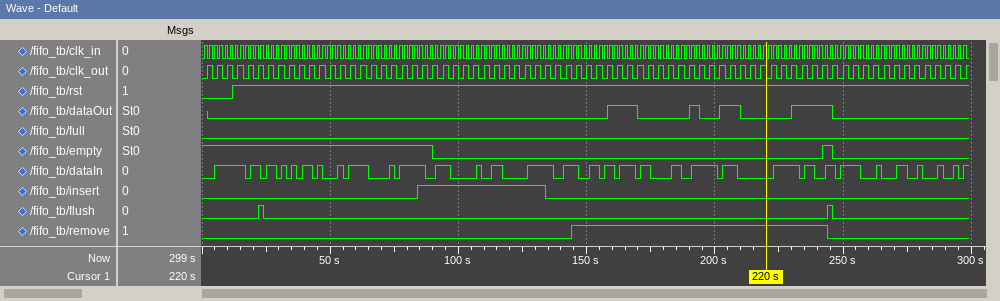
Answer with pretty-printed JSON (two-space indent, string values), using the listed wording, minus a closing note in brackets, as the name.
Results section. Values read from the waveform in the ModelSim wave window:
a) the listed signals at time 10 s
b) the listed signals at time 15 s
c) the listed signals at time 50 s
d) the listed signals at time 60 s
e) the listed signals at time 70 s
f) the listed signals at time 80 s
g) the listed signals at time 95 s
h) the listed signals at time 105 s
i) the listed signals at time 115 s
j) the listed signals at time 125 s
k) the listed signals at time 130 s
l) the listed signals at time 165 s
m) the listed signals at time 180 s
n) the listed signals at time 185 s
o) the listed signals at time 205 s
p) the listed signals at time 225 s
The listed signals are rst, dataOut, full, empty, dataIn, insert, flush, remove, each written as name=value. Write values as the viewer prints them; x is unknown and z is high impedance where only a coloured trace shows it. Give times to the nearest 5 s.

{
  "the listed signals at time 10 s": "rst=0, dataOut=0, full=0, empty=1, dataIn=1, insert=0, flush=0, remove=0",
  "the listed signals at time 15 s": "rst=1, dataOut=0, full=0, empty=1, dataIn=1, insert=0, flush=0, remove=0",
  "the listed signals at time 50 s": "rst=1, dataOut=0, full=0, empty=1, dataIn=0, insert=0, flush=0, remove=0",
  "the listed signals at time 60 s": "rst=1, dataOut=0, full=0, empty=1, dataIn=1, insert=0, flush=0, remove=0",
  "the listed signals at time 70 s": "rst=1, dataOut=0, full=0, empty=1, dataIn=0, insert=0, flush=0, remove=0",
  "the listed signals at time 80 s": "rst=1, dataOut=0, full=0, empty=1, dataIn=1, insert=0, flush=0, remove=0",
  "the listed signals at time 95 s": "rst=1, dataOut=0, full=0, empty=0, dataIn=1, insert=1, flush=0, remove=0",
  "the listed signals at time 105 s": "rst=1, dataOut=0, full=0, empty=0, dataIn=0, insert=1, flush=0, remove=0",
  "the listed signals at time 115 s": "rst=1, dataOut=0, full=0, empty=0, dataIn=1, insert=1, flush=0, remove=0",
  "the listed signals at time 125 s": "rst=1, dataOut=0, full=0, empty=0, dataIn=0, insert=1, flush=0, remove=0",
  "the listed signals at time 130 s": "rst=1, dataOut=0, full=0, empty=0, dataIn=1, insert=1, flush=0, remove=0",
  "the listed signals at time 165 s": "rst=1, dataOut=1, full=0, empty=0, dataIn=1, insert=0, flush=0, remove=1",
  "the listed signals at time 180 s": "rst=1, dataOut=0, full=0, empty=0, dataIn=0, insert=0, flush=0, remove=1",
  "the listed signals at time 185 s": "rst=1, dataOut=0, full=0, empty=0, dataIn=1, insert=0, flush=0, remove=1",
  "the listed signals at time 205 s": "rst=1, dataOut=1, full=0, empty=0, dataIn=1, insert=0, flush=0, remove=1",
  "the listed signals at time 225 s": "rst=1, dataOut=0, full=0, empty=0, dataIn=1, insert=0, flush=0, remove=1"
}
